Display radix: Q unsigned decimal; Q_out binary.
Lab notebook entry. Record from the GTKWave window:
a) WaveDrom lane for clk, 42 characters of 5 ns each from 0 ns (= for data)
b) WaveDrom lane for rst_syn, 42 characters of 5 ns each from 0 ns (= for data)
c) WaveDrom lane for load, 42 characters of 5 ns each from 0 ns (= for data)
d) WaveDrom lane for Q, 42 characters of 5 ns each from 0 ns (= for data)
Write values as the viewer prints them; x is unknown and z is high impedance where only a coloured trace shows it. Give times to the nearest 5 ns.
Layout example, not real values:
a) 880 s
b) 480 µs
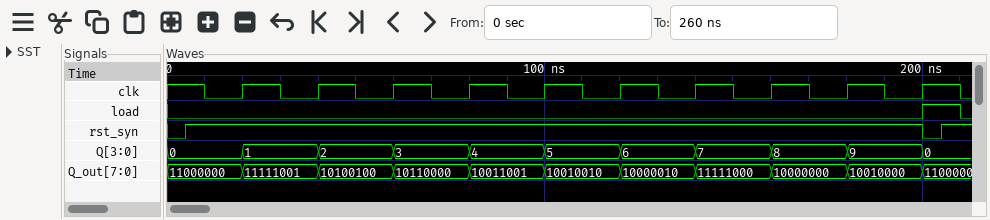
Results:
a) {name: 'clk', wave: '1.0.1.0.1.0.1.0.1.0.1.0.1.0.1.0.1.0.1.0.1.'}
b) {name: 'rst_syn', wave: '01......................................01'}
c) {name: 'load', wave: '0.......................................1.'}
d) {name: 'Q', wave: '=...=...=...=...=...=...=...=...=...=...=.', data: '0 1 2 3 4 5 6 7 8 9 0'}
